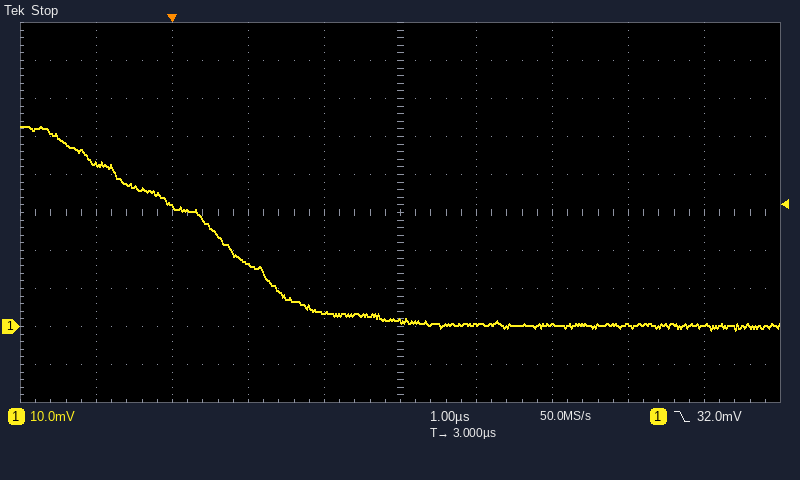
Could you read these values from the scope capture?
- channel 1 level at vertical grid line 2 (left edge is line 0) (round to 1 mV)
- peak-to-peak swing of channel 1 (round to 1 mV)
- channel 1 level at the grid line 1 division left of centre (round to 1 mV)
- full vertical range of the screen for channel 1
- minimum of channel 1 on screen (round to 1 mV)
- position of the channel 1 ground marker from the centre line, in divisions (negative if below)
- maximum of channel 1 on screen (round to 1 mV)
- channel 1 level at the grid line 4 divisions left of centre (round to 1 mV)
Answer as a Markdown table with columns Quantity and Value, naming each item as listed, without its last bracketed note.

| Quantity | Value |
|---|---|
| channel 1 level at vertical grid line 2 (left edge is line 0) | 32 mV |
| peak-to-peak swing of channel 1 | 54 mV |
| channel 1 level at the grid line 1 division left of centre | 4 mV |
| full vertical range of the screen for channel 1 | 100 mV |
| minimum of channel 1 on screen | -1 mV |
| position of the channel 1 ground marker from the centre line, in divisions | -3.0 div |
| maximum of channel 1 on screen | 53 mV |
| channel 1 level at the grid line 4 divisions left of centre | 43 mV |
